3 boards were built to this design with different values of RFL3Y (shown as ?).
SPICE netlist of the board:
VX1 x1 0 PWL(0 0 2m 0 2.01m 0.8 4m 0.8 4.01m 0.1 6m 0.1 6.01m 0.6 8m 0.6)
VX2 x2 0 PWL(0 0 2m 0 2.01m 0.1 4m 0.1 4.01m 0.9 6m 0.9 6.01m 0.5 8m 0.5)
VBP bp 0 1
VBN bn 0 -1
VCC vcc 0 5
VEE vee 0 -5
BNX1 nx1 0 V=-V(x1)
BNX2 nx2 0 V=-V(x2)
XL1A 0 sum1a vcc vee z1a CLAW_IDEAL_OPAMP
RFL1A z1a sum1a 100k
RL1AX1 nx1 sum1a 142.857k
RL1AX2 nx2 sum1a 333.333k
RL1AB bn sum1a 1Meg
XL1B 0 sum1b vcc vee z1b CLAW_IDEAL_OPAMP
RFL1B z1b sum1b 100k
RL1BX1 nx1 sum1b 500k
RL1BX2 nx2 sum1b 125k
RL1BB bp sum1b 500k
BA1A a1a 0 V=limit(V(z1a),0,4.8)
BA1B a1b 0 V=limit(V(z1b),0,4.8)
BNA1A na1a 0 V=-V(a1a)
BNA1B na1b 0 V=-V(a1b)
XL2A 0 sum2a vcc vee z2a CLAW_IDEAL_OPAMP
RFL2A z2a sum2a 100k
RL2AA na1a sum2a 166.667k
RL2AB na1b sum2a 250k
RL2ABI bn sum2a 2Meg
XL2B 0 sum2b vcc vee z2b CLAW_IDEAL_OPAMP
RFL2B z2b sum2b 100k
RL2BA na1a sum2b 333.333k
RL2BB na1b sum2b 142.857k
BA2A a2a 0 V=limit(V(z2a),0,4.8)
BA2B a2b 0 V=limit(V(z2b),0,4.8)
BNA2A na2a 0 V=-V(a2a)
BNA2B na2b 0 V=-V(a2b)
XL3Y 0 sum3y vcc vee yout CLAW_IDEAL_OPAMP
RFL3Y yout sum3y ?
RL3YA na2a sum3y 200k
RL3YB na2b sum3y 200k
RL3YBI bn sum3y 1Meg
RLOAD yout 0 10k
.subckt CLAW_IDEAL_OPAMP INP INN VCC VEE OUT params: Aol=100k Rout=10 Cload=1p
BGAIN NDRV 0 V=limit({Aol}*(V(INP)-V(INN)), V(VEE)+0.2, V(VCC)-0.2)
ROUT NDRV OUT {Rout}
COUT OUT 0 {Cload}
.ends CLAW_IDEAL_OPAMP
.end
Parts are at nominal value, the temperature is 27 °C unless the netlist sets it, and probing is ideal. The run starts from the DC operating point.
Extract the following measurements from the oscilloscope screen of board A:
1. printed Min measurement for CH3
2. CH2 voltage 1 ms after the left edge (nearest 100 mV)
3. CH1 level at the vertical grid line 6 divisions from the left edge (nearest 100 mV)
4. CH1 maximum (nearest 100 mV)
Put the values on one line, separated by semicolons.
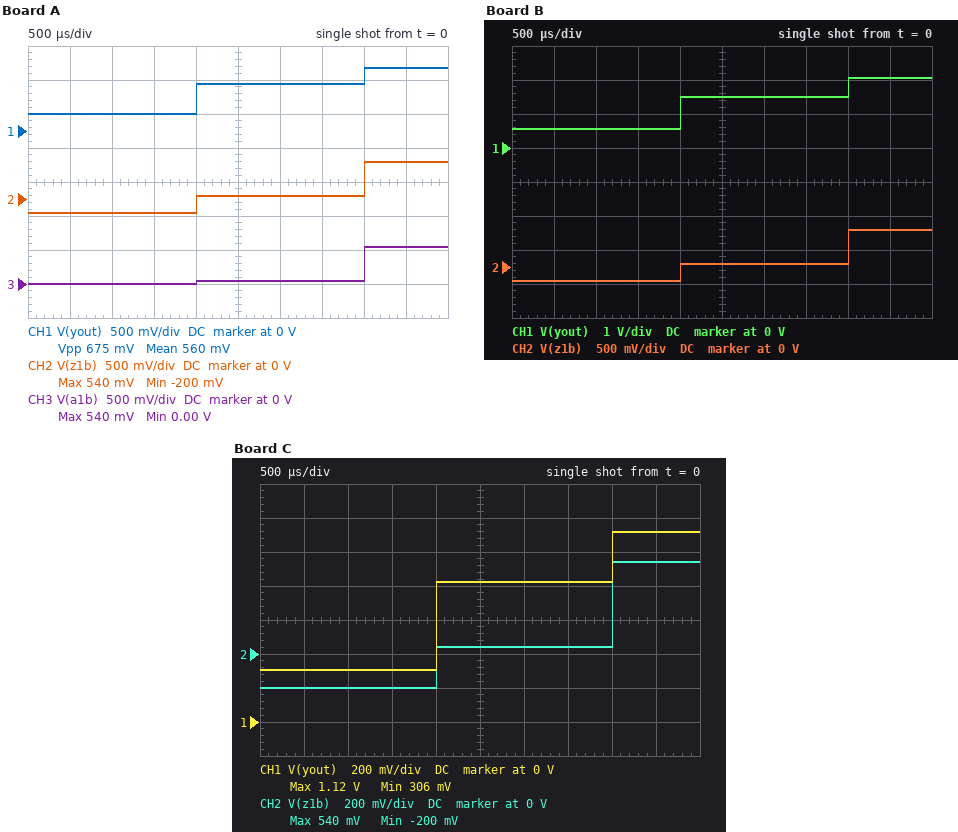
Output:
0.00 V; -200 mV; 700 mV; 900 mV
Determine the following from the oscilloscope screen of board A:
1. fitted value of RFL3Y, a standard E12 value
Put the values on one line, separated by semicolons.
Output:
150 kΩ
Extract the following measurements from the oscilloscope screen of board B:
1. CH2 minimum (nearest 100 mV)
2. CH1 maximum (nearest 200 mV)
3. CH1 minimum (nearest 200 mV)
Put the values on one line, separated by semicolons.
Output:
-200 mV; 2.0 V; 600 mV
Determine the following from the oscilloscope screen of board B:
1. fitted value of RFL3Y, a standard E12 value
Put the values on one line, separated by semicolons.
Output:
330 kΩ
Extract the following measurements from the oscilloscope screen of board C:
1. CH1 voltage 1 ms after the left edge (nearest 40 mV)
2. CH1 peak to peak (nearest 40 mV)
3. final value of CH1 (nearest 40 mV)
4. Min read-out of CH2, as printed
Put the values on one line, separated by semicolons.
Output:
320 mV; 800 mV; 1.12 V; -200 mV
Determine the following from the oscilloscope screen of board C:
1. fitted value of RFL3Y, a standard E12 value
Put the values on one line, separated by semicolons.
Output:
180 kΩ
